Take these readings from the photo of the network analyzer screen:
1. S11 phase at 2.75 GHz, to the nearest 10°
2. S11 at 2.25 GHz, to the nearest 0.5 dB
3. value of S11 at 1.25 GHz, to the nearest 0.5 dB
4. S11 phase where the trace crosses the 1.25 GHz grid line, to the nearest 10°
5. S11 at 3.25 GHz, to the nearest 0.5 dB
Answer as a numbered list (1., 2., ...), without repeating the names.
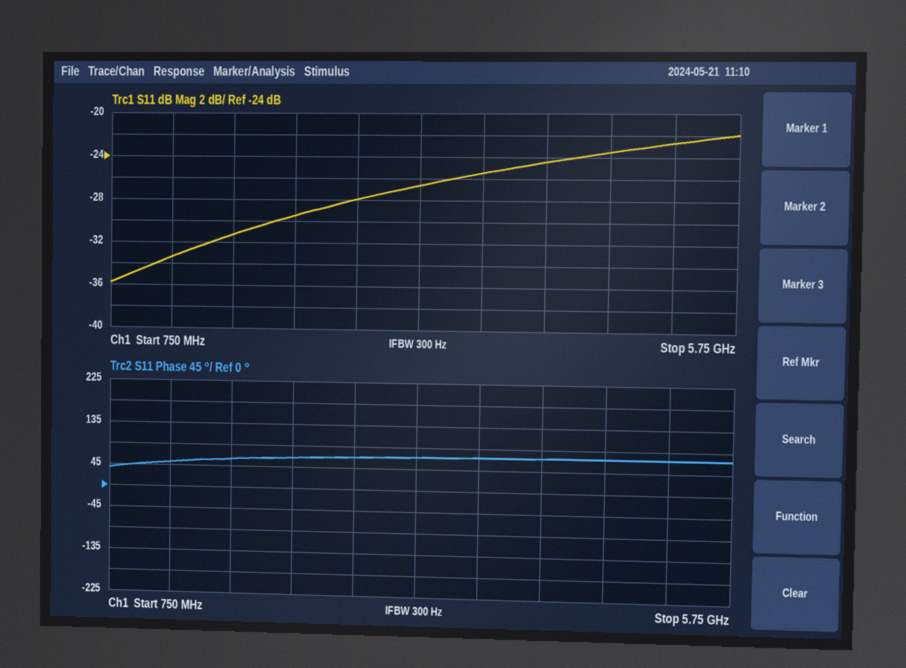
1. 70°
2. -29.5 dB
3. -33.5 dB
4. 50°
5. -26.5 dB
